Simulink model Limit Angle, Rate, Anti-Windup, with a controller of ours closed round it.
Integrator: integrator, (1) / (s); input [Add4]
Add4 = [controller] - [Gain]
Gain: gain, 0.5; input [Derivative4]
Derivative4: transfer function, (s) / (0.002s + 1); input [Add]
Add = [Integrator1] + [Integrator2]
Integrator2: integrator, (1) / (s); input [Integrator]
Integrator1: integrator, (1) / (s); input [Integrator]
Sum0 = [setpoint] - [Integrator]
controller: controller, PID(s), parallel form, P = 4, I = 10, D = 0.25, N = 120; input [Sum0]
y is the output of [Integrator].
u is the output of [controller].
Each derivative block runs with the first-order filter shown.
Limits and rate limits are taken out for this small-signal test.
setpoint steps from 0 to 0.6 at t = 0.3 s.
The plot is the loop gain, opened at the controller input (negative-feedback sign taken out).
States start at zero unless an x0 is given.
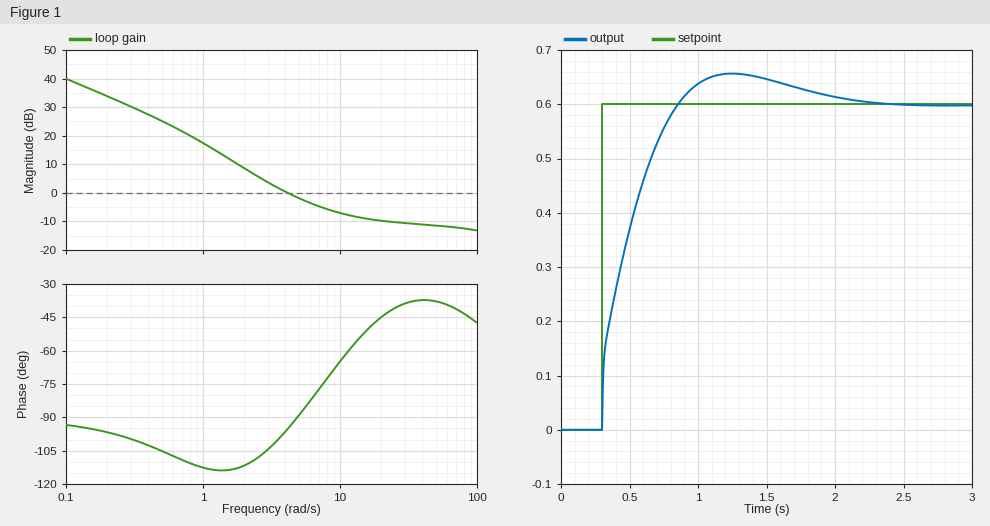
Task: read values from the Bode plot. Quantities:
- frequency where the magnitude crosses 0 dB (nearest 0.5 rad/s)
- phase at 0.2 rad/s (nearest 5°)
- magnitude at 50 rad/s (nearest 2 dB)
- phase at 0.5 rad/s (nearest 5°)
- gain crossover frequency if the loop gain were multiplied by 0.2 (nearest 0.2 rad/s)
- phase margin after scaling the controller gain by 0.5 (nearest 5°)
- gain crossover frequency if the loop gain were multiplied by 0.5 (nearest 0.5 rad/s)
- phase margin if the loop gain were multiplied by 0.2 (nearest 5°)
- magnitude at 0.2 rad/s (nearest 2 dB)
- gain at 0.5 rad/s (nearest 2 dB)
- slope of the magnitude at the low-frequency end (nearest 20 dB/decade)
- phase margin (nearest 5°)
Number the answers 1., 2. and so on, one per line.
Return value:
1. 4.0 rad/s
2. -95°
3. -12 dB
4. -105°
5. 1.4 rad/s
6. 70°
7. 2.5 rad/s
8. 65°
9. 34 dB
10. 26 dB
11. -20 dB/decade
12. 85°
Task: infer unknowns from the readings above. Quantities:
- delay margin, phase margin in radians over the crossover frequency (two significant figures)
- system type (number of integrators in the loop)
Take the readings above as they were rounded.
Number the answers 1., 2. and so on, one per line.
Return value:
1. 0.37 s
2. 1
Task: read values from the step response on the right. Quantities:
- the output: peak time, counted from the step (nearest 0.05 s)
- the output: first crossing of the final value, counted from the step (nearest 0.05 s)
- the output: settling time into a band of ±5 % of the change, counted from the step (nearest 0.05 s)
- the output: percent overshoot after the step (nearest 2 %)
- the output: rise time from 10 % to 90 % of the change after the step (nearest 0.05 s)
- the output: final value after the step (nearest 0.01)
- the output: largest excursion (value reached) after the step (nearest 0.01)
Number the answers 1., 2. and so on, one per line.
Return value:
1. 0.95 s
2. 0.55 s
3. 1.45 s
4. 10 %
5. 0.40 s
6. 0.60
7. 0.66
